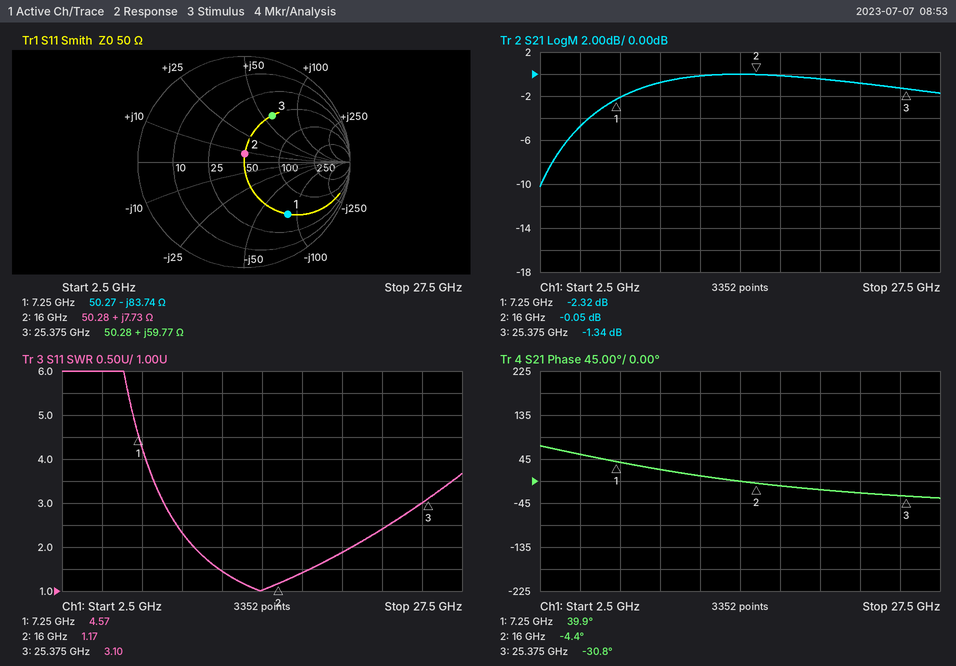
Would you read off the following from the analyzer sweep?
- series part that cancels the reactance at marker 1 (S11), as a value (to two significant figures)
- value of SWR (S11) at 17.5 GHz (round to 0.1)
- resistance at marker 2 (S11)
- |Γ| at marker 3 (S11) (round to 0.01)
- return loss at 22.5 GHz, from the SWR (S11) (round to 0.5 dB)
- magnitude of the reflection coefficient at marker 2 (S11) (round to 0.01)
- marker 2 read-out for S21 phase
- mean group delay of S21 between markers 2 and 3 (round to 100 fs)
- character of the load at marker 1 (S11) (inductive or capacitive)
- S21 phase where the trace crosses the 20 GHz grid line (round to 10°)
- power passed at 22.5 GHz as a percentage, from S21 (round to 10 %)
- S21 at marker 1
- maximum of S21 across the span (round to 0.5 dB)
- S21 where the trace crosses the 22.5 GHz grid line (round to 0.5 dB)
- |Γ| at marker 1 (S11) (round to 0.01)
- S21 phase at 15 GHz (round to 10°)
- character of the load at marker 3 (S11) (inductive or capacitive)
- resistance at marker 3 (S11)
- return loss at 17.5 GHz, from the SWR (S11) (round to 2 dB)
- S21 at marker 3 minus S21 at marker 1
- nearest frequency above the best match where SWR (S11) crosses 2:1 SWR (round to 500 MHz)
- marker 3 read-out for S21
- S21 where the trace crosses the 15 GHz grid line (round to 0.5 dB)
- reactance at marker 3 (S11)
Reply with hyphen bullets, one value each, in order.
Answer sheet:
- 1.8 nH
- 1.4
- 50.28 Ω
- 0.51
- 7.5 dB
- 0.08
- -4.4°
- 7.8 ps
- capacitive
- -20°
- 80 %
- -2.32 dB
- 0.0 dB
- -1.0 dB
- 0.64
- 0°
- inductive
- 50.28 Ω
- 16 dB
- 0.98 dB
- 20.5 GHz
- -1.34 dB
- 0.0 dB
- +59.77 Ω
